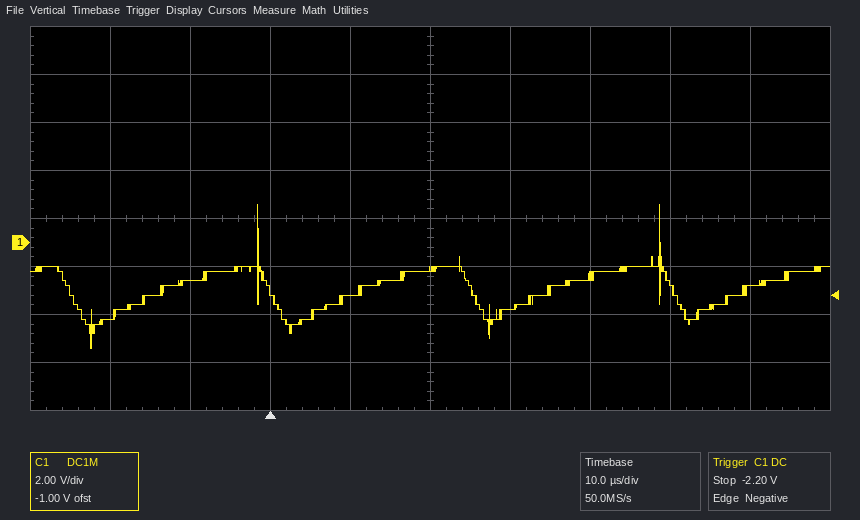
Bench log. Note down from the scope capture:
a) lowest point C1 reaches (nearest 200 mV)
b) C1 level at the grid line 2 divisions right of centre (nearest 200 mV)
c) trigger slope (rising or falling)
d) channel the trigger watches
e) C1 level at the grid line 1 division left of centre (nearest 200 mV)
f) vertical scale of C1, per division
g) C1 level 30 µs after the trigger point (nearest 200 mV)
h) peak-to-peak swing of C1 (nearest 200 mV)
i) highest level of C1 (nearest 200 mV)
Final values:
-4.4 V
-1.4 V
falling
C1
-2.2 V
2 V
-2.8 V
6.0 V
1.6 V
